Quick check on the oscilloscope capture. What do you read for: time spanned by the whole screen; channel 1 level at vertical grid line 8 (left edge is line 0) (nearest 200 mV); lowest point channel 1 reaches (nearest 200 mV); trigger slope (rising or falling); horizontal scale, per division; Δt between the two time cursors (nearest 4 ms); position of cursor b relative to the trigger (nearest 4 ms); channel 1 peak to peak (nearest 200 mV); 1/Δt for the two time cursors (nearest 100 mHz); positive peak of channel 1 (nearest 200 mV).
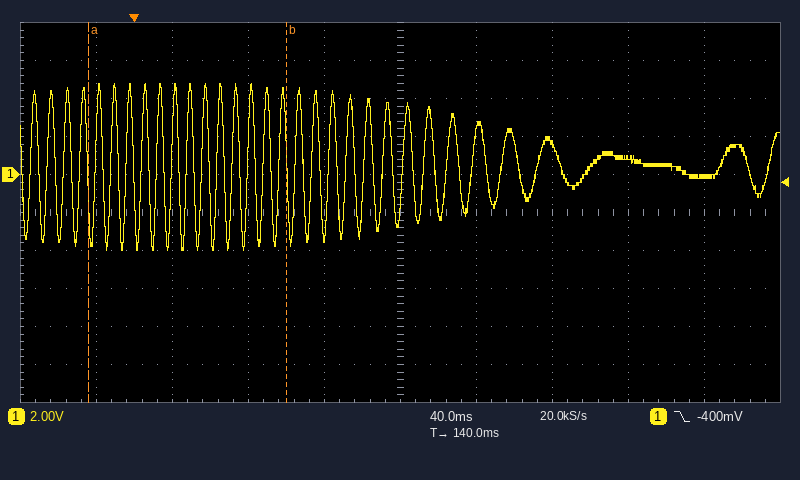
400 ms
800 mV
-4.0 V
falling
40 ms
104 ms
+80 ms
8.8 V
9.6 Hz
4.8 V
